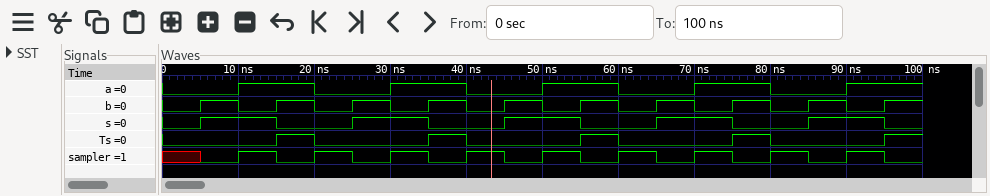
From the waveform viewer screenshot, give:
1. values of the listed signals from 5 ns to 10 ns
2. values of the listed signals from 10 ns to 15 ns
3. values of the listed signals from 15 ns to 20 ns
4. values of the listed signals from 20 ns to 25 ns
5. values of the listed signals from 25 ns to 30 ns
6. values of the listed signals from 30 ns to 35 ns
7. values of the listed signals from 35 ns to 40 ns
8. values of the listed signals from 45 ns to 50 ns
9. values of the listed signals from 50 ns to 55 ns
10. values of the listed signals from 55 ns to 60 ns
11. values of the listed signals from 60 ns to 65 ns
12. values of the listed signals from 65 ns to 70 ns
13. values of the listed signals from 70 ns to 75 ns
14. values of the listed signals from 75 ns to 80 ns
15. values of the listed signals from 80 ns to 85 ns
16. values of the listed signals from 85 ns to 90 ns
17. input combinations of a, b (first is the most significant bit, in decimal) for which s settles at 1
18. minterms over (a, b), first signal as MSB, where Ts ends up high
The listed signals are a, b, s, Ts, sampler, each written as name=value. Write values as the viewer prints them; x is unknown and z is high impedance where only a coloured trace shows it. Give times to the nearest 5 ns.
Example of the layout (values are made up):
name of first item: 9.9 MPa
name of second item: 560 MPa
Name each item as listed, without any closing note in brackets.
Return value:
values of the listed signals from 5 ns to 10 ns: a=0, b=1, s=1, Ts=0, sampler=0
values of the listed signals from 10 ns to 15 ns: a=1, b=0, s=1, Ts=0, sampler=1
values of the listed signals from 15 ns to 20 ns: a=1, b=1, s=0, Ts=1, sampler=0
values of the listed signals from 20 ns to 25 ns: a=0, b=0, s=0, Ts=0, sampler=1
values of the listed signals from 25 ns to 30 ns: a=0, b=1, s=1, Ts=0, sampler=0
values of the listed signals from 30 ns to 35 ns: a=1, b=0, s=1, Ts=0, sampler=1
values of the listed signals from 35 ns to 40 ns: a=1, b=1, s=0, Ts=1, sampler=0
values of the listed signals from 45 ns to 50 ns: a=0, b=1, s=1, Ts=0, sampler=0
values of the listed signals from 50 ns to 55 ns: a=1, b=0, s=1, Ts=0, sampler=1
values of the listed signals from 55 ns to 60 ns: a=1, b=1, s=0, Ts=1, sampler=0
values of the listed signals from 60 ns to 65 ns: a=0, b=0, s=0, Ts=0, sampler=1
values of the listed signals from 65 ns to 70 ns: a=0, b=1, s=1, Ts=0, sampler=0
values of the listed signals from 70 ns to 75 ns: a=1, b=0, s=1, Ts=0, sampler=1
values of the listed signals from 75 ns to 80 ns: a=1, b=1, s=0, Ts=1, sampler=0
values of the listed signals from 80 ns to 85 ns: a=0, b=0, s=0, Ts=0, sampler=1
values of the listed signals from 85 ns to 90 ns: a=0, b=1, s=1, Ts=0, sampler=0
input combinations of a, b (first is the most significant bit, in decimal) for which s settles at 1: 1, 2
minterms over (a, b), first signal as MSB, where Ts ends up high: 3
